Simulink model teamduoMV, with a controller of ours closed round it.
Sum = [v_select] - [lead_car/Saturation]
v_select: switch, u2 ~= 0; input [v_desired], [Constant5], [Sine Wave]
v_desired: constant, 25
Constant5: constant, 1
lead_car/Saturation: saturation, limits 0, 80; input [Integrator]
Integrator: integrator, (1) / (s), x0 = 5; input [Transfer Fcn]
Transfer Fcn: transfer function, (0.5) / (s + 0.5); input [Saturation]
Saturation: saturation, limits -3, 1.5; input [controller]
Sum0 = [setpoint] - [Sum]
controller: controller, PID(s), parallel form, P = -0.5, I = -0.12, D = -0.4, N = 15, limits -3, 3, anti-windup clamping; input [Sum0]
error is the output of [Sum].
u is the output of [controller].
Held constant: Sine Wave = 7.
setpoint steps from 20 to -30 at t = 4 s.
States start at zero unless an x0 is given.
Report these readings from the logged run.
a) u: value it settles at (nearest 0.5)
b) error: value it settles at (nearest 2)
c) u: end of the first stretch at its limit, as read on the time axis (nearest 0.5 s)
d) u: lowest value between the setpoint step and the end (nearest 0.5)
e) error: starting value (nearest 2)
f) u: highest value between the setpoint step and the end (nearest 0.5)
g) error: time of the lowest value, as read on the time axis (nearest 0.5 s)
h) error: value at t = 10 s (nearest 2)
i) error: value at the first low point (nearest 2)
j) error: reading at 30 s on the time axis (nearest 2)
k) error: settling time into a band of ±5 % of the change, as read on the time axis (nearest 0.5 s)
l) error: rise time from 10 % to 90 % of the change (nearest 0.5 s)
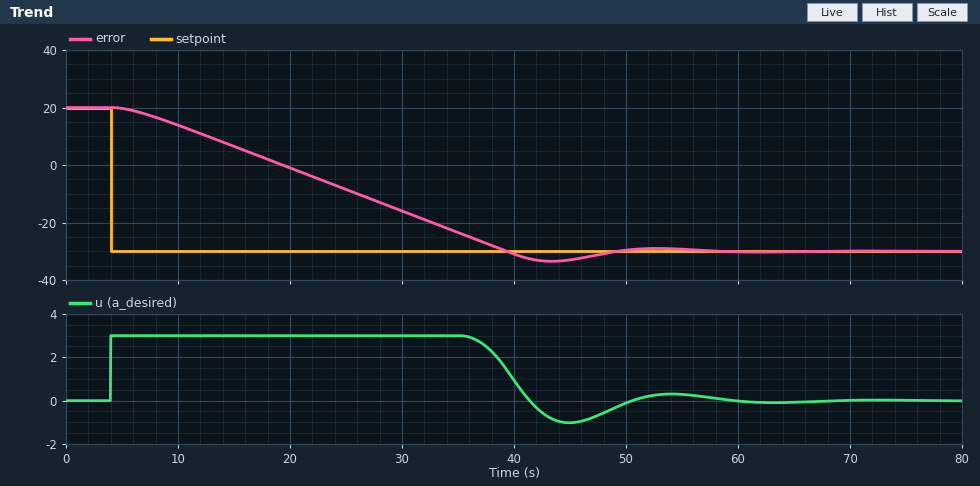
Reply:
0.0
-30
36.0 s
-1.0
20
3.0
43.5 s
14
-34
-16
46.0 s
27.0 s
